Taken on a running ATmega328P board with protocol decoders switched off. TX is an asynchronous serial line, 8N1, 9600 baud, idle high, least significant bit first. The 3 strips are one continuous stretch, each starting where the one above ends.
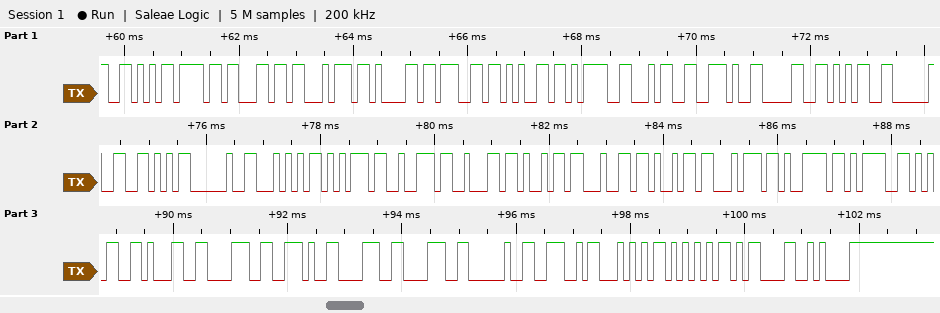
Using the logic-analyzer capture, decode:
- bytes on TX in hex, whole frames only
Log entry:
0x56 0x6F 0x6C 0x74 0x61 0x67 0x65 0x3D 0x34 0x2E 0x30 0x35 0x20 0x56 0x20 0x54 0x75 0x72 0x62 0x69 0x64 0x69 0x74 0x79 0x3D 0x35 0x31 0x38 0x2E 0x38 0x38 0x20 0x4E 0x54 0x55 0x0D 0x0A
